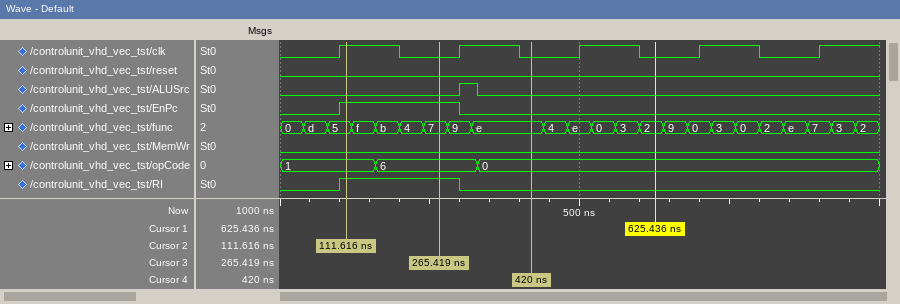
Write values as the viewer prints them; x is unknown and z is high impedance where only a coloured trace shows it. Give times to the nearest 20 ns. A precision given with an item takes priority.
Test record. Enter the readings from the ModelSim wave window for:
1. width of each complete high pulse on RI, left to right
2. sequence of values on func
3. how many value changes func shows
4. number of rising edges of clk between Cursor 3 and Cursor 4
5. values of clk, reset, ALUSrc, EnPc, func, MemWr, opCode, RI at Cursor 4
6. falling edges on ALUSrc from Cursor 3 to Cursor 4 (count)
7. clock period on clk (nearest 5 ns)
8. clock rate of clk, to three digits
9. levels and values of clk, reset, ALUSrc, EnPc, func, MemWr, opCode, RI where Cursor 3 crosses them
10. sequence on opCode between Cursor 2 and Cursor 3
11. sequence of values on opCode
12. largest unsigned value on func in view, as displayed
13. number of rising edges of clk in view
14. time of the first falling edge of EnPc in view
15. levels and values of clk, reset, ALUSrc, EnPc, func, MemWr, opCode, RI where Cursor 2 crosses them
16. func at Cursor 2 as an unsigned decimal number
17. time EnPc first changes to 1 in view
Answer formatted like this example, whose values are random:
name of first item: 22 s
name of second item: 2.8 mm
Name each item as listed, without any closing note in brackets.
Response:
width of each complete high pulse on RI, left to right: 200 ns
sequence of values on func: 0, d, 5, f, b, 4, 7, 9, e, 4, e, 0, 3, 2, 9, 0, 3, 0, 2, e, 7, 3, 2
how many value changes func shows: 22
number of rising edges of clk between Cursor 3 and Cursor 4: 1
values of clk, reset, ALUSrc, EnPc, func, MemWr, opCode, RI at Cursor 4: clk=0, reset=0, ALUSrc=0, EnPc=0, func=e, MemWr=0, opCode=0, RI=0
falling edges on ALUSrc from Cursor 3 to Cursor 4: 1
clock period on clk: 200 ns
clock rate of clk, to three digits: 5.00 MHz
levels and values of clk, reset, ALUSrc, EnPc, func, MemWr, opCode, RI where Cursor 3 crosses them: clk=0, reset=0, ALUSrc=0, EnPc=1, func=7, MemWr=0, opCode=6, RI=1
sequence on opCode between Cursor 2 and Cursor 3: 1, 6
sequence of values on opCode: 1, 6, 0
largest unsigned value on func in view, as displayed: f
number of rising edges of clk in view: 5
time of the first falling edge of EnPc in view: 300 ns
levels and values of clk, reset, ALUSrc, EnPc, func, MemWr, opCode, RI where Cursor 2 crosses them: clk=1, reset=0, ALUSrc=0, EnPc=1, func=5, MemWr=0, opCode=1, RI=1
func at Cursor 2 as an unsigned decimal number: 5
time EnPc first changes to 1 in view: 100 ns
